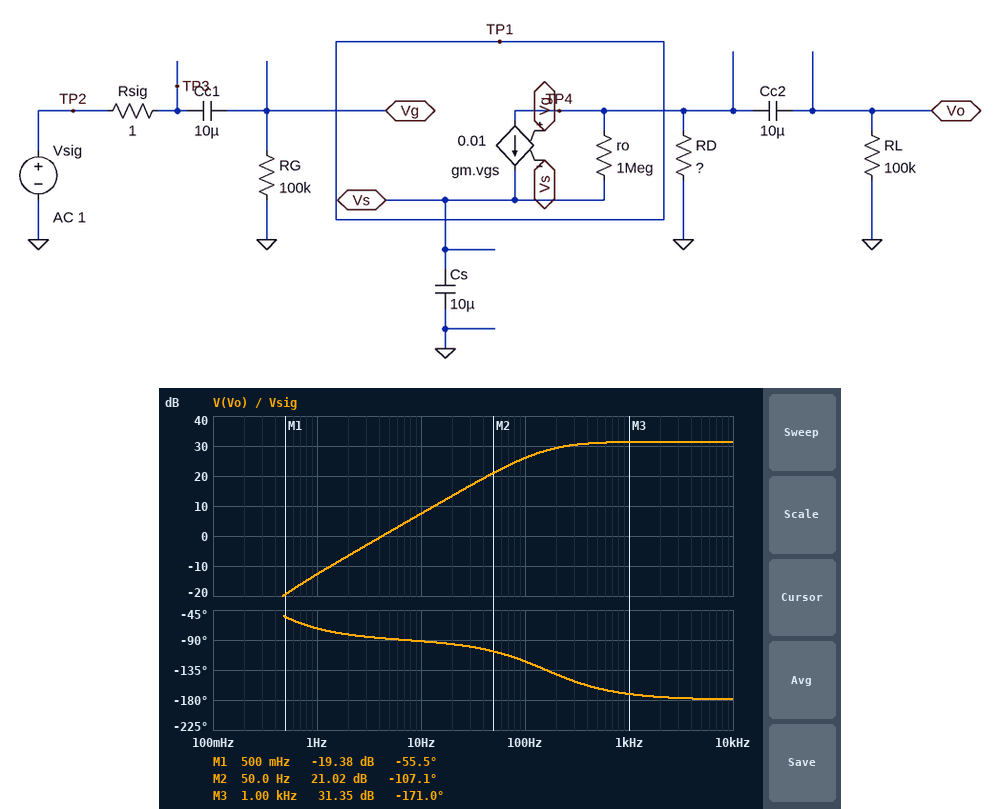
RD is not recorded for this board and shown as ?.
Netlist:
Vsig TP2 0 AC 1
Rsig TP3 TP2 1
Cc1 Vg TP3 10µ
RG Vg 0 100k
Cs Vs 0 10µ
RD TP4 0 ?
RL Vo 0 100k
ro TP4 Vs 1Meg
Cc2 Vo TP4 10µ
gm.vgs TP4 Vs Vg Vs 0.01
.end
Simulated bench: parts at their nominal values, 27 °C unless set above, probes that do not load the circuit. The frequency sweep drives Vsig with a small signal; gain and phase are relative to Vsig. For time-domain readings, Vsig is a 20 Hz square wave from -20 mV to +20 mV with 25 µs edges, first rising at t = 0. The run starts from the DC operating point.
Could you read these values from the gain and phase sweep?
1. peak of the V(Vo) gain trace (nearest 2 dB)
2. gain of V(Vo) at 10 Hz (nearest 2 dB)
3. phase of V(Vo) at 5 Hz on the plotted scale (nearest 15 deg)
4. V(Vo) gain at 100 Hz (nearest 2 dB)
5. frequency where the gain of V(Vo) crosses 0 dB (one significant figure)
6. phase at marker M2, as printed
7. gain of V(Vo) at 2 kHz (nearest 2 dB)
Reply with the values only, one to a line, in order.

32 dB
8 dB
-90 deg
26 dB
4 Hz
-107.1 deg
32 dB
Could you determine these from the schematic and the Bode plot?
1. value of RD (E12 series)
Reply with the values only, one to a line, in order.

3.9 kΩ
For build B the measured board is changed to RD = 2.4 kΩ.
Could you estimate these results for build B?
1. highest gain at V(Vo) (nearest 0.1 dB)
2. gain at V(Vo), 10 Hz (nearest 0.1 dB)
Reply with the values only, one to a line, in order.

27.4 dB
3.3 dB
